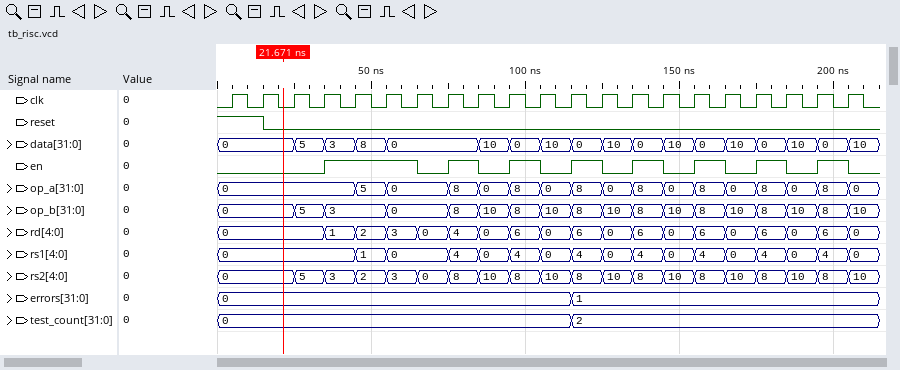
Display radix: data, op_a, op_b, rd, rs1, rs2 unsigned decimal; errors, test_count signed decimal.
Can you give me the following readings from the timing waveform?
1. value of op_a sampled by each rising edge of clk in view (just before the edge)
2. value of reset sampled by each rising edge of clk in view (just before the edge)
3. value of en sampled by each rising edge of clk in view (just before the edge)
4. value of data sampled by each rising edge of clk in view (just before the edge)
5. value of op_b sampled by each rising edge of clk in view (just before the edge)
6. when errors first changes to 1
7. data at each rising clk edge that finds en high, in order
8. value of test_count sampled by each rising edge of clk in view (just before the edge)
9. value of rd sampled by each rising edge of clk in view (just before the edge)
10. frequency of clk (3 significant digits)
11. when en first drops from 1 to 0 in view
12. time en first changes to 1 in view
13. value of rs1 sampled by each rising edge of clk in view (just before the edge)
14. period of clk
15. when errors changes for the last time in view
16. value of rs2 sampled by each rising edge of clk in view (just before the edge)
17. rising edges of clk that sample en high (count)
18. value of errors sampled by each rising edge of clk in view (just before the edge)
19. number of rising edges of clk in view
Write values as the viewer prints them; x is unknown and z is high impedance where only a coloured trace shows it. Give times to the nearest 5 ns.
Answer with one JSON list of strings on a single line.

["0, 0, 0, 0, 0, 5, 0, 0, 8, 0, 8, 0, 8, 0, 8, 0, 8, 0, 8, 0, 8", "1 1 0 0 0 0 0 0 0 0 0 0 0 0 0 0 0 0 0 0 0", "0 0 0 0 1 1 1 0 1 0 1 0 1 0 1 0 1 0 1 0 1", "0, 0, 0, 5, 3, 8, 0, 0, 0, 10, 0, 10, 0, 10, 0, 10, 0, 10, 0, 10, 0", "0, 0, 0, 5, 3, 3, 0, 0, 8, 10, 8, 10, 8, 10, 8, 10, 8, 10, 8, 10, 8", "115 ns", "3, 8, 0, 0, 0, 0, 0, 0, 0, 0", "0, 0, 0, 0, 0, 0, 0, 0, 0, 0, 0, 0, 2, 2, 2, 2, 2, 2, 2, 2, 2", "0, 0, 0, 0, 1, 2, 3, 0, 4, 0, 6, 0, 6, 0, 6, 0, 6, 0, 6, 0, 6", "100 MHz", "65 ns", "35 ns", "0, 0, 0, 0, 0, 1, 0, 0, 4, 0, 4, 0, 4, 0, 4, 0, 4, 0, 4, 0, 4", "10 ns", "115 ns", "0, 0, 0, 5, 3, 2, 3, 0, 8, 10, 8, 10, 8, 10, 8, 10, 8, 10, 8, 10, 8", "10", "0, 0, 0, 0, 0, 0, 0, 0, 0, 0, 0, 0, 1, 1, 1, 1, 1, 1, 1, 1, 1", "21"]
